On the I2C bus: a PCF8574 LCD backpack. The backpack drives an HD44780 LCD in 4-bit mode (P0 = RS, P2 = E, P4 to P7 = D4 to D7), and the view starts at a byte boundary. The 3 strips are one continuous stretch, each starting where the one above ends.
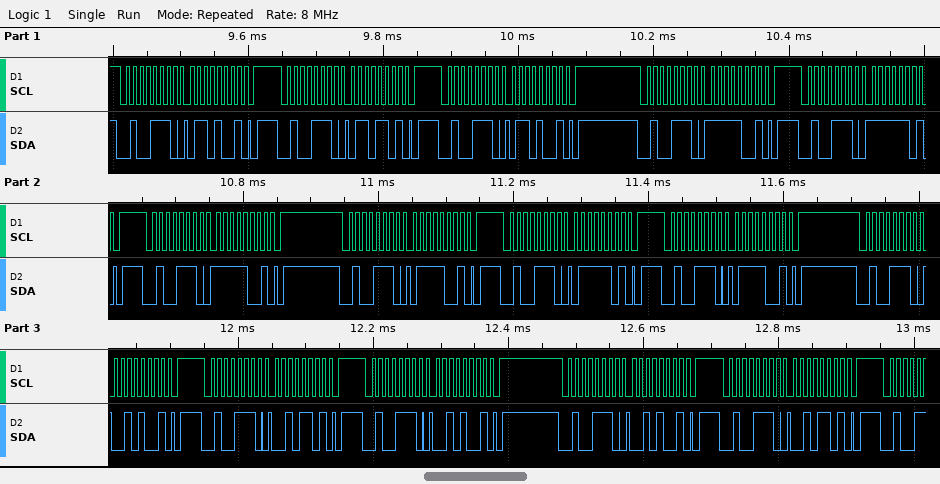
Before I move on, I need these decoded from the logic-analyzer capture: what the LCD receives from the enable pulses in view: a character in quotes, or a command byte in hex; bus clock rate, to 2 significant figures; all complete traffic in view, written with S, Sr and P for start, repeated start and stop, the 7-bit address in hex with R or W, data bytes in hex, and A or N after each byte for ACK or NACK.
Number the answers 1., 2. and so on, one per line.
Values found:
1. 'o' 'r'
2. 100 kHz
3. S 27W A 69 A P S 27W A 6D A P S 27W A 69 A P S 27W A F9 A P S 27W A FD A P S 27W A F9 A P S 27W A 79 A P S 27W A 7D A P S 27W A 79 A P S 27W A 29 A P S 27W A 2D A P S 27W A 29 A P S 27W A 29 A P S 27W A 2D A P
